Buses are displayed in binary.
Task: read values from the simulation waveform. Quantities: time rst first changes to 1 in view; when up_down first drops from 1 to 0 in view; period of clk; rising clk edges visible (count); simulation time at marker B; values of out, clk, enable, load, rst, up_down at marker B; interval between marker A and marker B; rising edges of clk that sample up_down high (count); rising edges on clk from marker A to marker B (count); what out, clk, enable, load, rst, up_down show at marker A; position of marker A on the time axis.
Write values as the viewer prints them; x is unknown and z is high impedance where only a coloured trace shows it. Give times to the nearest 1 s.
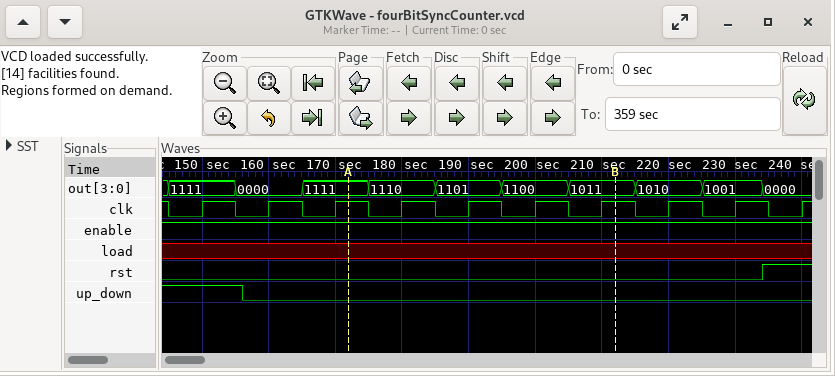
234 s
156 s
10 s
10
212 s
out=1011, clk=1, enable=1, load=x, rst=0, up_down=0
40 s
1
4
out=1111, clk=1, enable=1, load=x, rst=0, up_down=0
172 s
